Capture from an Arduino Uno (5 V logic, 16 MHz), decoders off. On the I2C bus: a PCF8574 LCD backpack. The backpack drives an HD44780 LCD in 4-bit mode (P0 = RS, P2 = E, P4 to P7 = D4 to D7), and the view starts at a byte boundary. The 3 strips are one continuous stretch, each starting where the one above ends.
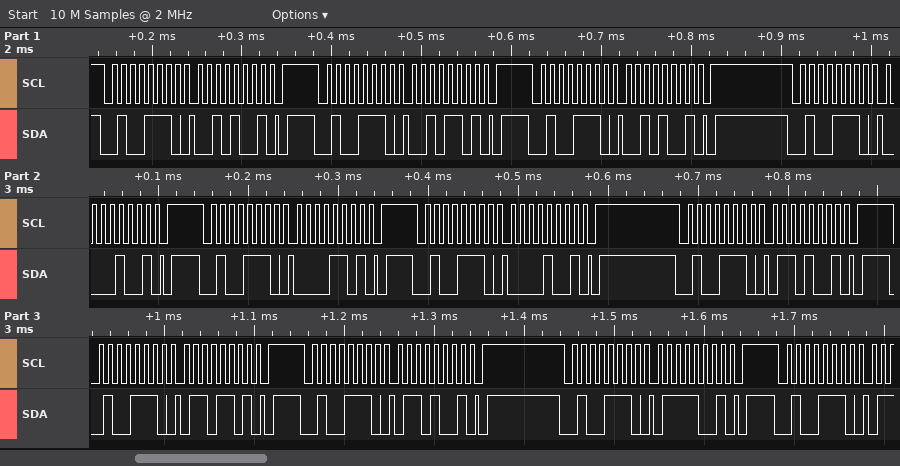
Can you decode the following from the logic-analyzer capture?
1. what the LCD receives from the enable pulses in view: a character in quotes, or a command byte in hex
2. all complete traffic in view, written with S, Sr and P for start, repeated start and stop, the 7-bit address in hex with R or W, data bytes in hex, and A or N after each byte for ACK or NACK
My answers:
' '
S 27W A 29 A P S 27W A 2D A P S 27W A 29 A P S 27W A 09 A P S 27W A 0D A P S 27W A 09 A P S 27W A 69 A P S 27W A 6D A P S 27W A 69 A P S 27W A 79 A P S 27W A
